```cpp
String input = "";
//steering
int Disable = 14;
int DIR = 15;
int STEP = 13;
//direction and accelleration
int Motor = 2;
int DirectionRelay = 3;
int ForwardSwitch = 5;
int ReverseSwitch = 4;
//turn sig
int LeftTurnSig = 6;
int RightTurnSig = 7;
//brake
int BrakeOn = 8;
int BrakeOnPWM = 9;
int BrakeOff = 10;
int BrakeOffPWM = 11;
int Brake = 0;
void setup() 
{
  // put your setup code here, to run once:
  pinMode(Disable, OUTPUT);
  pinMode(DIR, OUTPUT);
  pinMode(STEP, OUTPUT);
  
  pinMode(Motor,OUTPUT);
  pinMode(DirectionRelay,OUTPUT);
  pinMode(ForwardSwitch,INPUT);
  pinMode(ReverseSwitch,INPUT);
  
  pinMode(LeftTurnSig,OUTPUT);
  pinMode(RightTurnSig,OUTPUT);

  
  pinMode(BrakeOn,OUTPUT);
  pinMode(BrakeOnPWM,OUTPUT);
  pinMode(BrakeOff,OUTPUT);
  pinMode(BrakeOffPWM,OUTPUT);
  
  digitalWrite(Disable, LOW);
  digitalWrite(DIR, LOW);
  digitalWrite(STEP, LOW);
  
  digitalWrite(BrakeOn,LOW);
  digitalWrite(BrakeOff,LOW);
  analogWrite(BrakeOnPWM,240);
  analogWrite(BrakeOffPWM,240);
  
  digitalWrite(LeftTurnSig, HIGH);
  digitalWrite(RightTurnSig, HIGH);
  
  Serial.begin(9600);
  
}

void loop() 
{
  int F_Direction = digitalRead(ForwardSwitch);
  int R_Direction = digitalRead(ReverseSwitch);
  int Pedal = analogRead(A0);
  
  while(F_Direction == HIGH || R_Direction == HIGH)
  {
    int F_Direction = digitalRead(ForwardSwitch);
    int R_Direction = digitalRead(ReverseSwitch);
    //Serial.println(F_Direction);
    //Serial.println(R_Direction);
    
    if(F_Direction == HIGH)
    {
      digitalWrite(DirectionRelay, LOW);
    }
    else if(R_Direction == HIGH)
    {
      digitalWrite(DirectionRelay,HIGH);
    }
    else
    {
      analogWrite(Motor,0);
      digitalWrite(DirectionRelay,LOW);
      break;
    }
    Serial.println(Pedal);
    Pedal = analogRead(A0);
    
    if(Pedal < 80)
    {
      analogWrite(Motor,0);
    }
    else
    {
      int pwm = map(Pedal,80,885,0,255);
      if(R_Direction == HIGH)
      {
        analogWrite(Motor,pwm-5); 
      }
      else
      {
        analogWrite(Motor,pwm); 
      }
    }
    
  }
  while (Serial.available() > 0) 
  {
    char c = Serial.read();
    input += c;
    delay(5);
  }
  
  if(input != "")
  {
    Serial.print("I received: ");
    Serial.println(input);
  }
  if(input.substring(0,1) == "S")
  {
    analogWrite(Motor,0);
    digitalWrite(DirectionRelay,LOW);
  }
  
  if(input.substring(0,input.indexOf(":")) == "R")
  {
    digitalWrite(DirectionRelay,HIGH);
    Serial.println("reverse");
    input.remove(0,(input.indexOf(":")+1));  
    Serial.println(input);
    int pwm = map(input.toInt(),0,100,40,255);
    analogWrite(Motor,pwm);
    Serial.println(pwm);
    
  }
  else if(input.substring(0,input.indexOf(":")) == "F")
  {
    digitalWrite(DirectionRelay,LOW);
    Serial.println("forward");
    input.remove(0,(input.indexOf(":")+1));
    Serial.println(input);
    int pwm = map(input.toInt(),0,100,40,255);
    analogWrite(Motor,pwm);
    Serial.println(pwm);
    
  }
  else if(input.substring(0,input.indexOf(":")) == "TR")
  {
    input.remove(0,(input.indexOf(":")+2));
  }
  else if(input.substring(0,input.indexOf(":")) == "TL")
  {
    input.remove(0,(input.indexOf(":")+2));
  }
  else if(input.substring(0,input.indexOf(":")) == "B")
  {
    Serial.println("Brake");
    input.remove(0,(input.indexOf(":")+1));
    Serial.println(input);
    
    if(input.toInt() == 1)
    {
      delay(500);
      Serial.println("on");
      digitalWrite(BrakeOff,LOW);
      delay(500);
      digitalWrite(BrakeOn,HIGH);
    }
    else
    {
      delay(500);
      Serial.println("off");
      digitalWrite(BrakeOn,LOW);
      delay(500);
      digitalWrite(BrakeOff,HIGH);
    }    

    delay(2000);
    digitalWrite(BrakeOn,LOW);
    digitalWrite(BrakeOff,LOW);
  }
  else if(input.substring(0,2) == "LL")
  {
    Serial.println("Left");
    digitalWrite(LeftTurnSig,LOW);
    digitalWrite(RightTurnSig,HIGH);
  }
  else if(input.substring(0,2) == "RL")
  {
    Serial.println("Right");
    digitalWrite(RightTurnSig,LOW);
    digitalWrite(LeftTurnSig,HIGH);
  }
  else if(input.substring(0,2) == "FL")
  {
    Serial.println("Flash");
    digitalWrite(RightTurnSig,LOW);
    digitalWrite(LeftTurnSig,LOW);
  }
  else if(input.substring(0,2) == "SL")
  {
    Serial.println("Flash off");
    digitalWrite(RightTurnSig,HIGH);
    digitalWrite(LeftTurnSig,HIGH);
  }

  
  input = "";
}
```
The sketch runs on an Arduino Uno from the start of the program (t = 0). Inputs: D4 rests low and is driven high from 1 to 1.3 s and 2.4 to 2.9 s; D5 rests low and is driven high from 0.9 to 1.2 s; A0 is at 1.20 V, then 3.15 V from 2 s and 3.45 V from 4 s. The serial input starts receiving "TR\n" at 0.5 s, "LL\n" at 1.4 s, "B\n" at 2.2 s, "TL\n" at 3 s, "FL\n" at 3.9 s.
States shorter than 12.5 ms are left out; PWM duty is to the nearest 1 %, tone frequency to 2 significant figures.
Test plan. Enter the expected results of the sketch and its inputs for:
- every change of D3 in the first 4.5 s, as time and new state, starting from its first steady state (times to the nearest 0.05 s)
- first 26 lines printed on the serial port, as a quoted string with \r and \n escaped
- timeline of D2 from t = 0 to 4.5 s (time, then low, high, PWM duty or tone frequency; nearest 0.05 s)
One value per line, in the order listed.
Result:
0 s low; 1.2 s high; 1.3 s low; 2.4 s high; 2.9 s low
"I received: TR\n\r\n245\r\n245\r\n245\r\n245\r\n245\r\n245\r\n245\r\n245\r\n245\r\n245\r\n245\r\n245\r\n245\r\n245\r\n245\r\n245\r\n245\r\n245\r\n245\r\n245\r\n245\r\n245\r\n245\r\n245\r\n"
0 s low; 2.4 s high; 2.9 s low
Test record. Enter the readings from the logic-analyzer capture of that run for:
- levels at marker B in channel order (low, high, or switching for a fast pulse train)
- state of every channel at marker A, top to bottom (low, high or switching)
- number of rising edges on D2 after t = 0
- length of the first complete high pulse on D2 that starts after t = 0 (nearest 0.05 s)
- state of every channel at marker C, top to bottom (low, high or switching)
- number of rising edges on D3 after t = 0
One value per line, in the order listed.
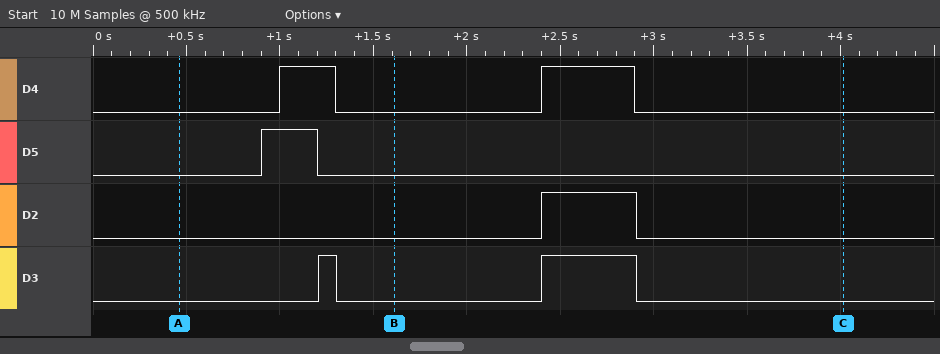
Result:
D4 low, D5 low, D2 low, D3 low
D4 low, D5 low, D2 low, D3 low
1
0.50 s
D4 low, D5 low, D2 low, D3 low
2
